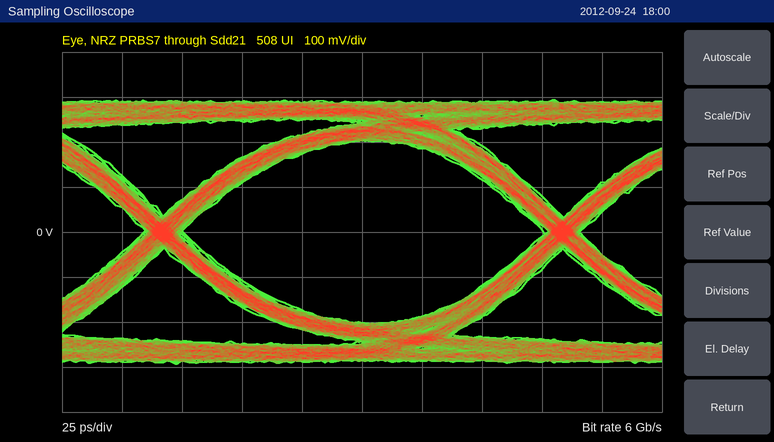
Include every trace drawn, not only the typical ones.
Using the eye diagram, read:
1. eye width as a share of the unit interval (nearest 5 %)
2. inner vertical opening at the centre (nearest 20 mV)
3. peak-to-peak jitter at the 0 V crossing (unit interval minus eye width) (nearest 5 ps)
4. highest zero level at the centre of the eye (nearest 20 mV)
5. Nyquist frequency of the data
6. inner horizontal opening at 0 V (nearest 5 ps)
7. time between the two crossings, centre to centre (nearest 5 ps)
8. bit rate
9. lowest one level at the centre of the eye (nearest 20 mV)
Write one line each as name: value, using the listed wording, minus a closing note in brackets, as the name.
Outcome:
eye width as a share of the unit interval: 90 %
inner vertical opening at the centre: 400 mV
peak-to-peak jitter at the 0 V crossing (unit interval minus eye width): 15 ps
highest zero level at the centre of the eye: -200 mV
Nyquist frequency of the data: 3 GHz
inner horizontal opening at 0 V: 150 ps
time between the two crossings, centre to centre: 165 ps
bit rate: 6 Gb/s
lowest one level at the centre of the eye: 200 mV
